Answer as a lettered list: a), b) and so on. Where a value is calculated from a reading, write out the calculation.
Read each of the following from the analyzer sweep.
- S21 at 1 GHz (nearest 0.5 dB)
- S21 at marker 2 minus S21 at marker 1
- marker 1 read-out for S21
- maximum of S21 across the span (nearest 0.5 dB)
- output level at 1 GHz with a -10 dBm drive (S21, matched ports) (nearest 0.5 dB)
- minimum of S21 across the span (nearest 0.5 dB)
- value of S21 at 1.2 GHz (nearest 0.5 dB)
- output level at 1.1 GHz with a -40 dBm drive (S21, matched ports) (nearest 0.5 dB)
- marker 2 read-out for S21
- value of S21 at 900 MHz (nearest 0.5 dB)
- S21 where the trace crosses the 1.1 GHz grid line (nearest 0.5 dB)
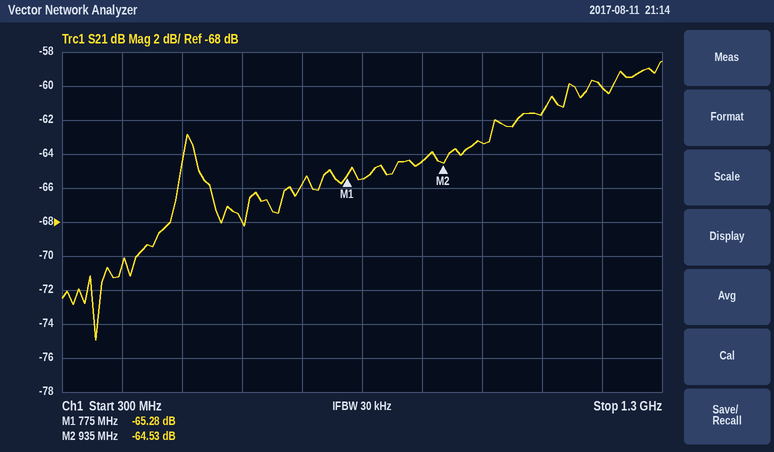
a) -63.5 dB
b) -64.53 − (-65.28) = 0.75 dB
c) -65.28 dB
d) -58.5 dB
e) -10 dBm + (-63.5 dB) = -73.5 dBm
f) -75.0 dB
g) -60.0 dB
h) -40 dBm + (-61.5 dB) = -101.5 dBm
i) -64.53 dB
j) -64.5 dB
k) -61.5 dB
